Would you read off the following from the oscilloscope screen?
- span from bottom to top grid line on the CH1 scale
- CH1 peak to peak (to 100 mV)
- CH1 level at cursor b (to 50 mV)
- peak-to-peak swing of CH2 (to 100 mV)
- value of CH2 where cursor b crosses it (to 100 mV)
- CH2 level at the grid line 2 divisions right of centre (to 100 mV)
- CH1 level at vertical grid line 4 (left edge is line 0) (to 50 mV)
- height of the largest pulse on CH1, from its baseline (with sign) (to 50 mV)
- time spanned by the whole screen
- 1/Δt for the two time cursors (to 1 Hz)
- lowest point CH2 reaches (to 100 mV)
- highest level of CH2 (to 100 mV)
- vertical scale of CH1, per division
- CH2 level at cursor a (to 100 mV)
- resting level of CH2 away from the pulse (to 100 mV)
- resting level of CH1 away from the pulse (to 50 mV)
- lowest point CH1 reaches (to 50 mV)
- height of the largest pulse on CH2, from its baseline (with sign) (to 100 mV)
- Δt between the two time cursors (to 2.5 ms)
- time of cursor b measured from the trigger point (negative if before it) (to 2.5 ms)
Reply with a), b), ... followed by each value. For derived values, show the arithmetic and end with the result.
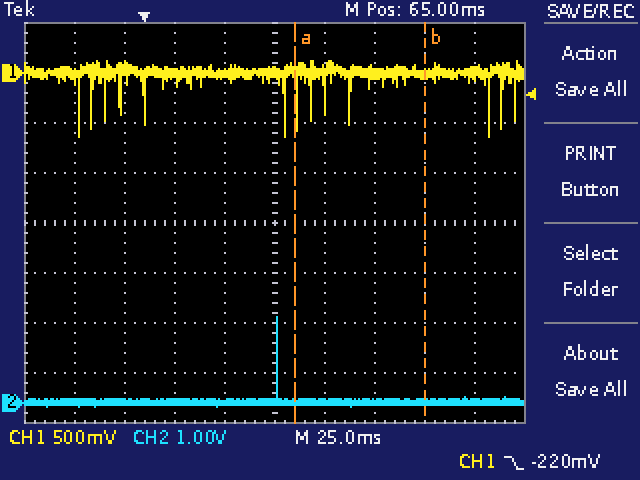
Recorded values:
a) 4 V
b) 800 mV
c) 0 mV
d) 1.7 V − (-100 mV) = 1.8 V
e) 0.0 V
f) 0.0 V
g) 0 mV
h) -650 mV − (0 mV) = -650 mV
i) 250 ms
j) 1 / 65.0 ms ≈ 15 Hz
k) -100 mV
l) 1.7 V
m) 500 mV
n) 0.0 V
o) 0.0 V
p) 0 mV
q) -650 mV
r) 1.7 V − (0.0 V) = +1.7 V
s) 65.0 ms
t) +140.0 ms
